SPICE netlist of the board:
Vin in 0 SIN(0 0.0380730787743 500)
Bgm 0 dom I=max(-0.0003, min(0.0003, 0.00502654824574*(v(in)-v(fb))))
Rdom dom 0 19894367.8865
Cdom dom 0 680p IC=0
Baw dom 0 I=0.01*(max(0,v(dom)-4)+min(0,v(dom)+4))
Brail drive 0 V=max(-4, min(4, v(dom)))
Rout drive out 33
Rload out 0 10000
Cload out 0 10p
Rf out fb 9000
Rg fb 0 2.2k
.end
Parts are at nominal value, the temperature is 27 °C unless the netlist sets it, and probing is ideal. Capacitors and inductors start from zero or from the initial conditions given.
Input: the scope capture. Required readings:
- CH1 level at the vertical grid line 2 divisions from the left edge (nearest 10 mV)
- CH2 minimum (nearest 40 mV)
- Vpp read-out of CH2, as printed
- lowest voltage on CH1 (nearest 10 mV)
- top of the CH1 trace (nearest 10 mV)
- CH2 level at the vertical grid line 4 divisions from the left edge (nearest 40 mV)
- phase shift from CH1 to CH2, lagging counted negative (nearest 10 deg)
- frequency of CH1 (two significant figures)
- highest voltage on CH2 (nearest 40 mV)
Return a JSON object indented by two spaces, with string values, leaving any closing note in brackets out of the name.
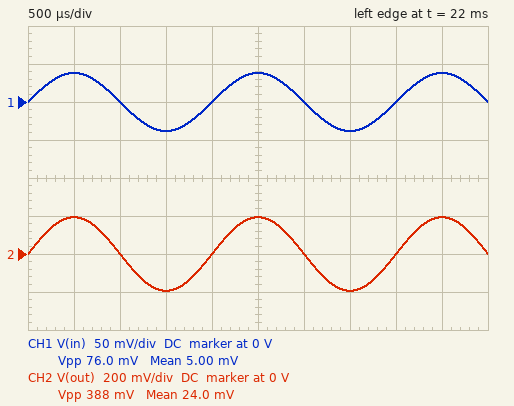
{
  "CH1 level at the vertical grid line 2 divisions from the left edge": "0 V",
  "CH2 minimum": "-200 mV",
  "Vpp read-out of CH2, as printed": "388 mV",
  "lowest voltage on CH1": "-40 mV",
  "top of the CH1 trace": "40 mV",
  "CH2 level at the vertical grid line 4 divisions from the left edge": "0 V",
  "phase shift from CH1 to CH2, lagging counted negative": "0 deg",
  "frequency of CH1": "500 Hz",
  "highest voltage on CH2": "200 mV"
}
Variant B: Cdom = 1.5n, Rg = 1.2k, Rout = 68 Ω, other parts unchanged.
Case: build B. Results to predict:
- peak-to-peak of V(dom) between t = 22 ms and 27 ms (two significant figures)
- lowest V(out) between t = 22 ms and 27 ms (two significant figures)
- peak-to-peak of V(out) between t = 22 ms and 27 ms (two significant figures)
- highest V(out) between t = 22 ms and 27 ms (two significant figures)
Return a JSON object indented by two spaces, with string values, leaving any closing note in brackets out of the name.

{
  "peak-to-peak of V(dom) between t = 22 ms and 27 ms": "660 mV",
  "lowest V(out) between t = 22 ms and 27 ms": "-320 mV",
  "peak-to-peak of V(out) between t = 22 ms and 27 ms": "650 mV",
  "highest V(out) between t = 22 ms and 27 ms": "320 mV"
}
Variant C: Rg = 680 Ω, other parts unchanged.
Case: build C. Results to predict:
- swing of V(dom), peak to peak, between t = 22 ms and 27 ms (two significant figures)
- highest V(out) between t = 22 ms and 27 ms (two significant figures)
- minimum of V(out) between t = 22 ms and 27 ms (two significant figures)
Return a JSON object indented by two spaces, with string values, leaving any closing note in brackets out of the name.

{
  "swing of V(dom), peak to peak, between t = 22 ms and 27 ms": "1.1 V",
  "highest V(out) between t = 22 ms and 27 ms": "540 mV",
  "minimum of V(out) between t = 22 ms and 27 ms": "-540 mV"
}
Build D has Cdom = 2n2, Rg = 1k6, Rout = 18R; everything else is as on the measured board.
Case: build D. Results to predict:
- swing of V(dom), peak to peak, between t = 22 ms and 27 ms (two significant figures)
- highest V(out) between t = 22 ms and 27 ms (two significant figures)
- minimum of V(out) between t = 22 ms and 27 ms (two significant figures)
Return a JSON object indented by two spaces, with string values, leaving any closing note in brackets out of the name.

{
  "swing of V(dom), peak to peak, between t = 22 ms and 27 ms": "510 mV",
  "highest V(out) between t = 22 ms and 27 ms": "250 mV",
  "minimum of V(out) between t = 22 ms and 27 ms": "-250 mV"
}
